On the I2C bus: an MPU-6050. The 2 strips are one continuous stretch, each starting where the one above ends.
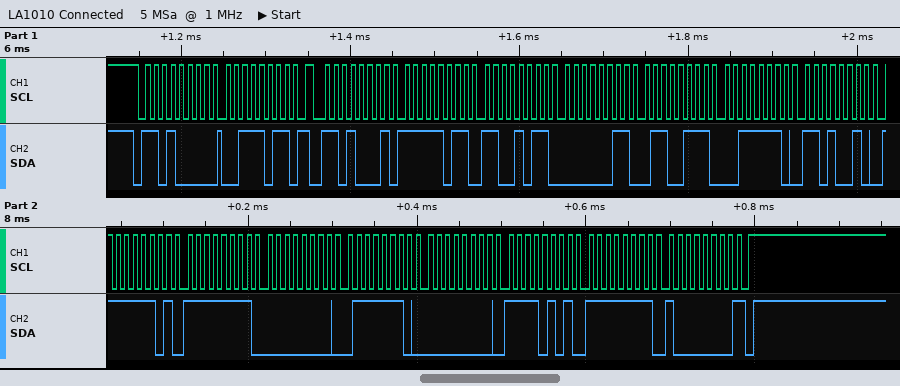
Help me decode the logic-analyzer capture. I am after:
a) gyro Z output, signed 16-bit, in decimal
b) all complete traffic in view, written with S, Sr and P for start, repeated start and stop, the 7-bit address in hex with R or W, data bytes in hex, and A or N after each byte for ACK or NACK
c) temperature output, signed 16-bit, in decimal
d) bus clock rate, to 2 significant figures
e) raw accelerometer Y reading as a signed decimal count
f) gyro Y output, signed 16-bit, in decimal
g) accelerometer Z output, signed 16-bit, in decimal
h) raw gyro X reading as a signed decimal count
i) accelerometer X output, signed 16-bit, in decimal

-128
S 68W A 3B A Sr 68R A FB A CB A 03 A 67 A 3E A D2 A FD A FF A 00 A 7E A 00 A F5 A FF A 80 N P
-513
100 kHz
871
245
16082
126
-1077
